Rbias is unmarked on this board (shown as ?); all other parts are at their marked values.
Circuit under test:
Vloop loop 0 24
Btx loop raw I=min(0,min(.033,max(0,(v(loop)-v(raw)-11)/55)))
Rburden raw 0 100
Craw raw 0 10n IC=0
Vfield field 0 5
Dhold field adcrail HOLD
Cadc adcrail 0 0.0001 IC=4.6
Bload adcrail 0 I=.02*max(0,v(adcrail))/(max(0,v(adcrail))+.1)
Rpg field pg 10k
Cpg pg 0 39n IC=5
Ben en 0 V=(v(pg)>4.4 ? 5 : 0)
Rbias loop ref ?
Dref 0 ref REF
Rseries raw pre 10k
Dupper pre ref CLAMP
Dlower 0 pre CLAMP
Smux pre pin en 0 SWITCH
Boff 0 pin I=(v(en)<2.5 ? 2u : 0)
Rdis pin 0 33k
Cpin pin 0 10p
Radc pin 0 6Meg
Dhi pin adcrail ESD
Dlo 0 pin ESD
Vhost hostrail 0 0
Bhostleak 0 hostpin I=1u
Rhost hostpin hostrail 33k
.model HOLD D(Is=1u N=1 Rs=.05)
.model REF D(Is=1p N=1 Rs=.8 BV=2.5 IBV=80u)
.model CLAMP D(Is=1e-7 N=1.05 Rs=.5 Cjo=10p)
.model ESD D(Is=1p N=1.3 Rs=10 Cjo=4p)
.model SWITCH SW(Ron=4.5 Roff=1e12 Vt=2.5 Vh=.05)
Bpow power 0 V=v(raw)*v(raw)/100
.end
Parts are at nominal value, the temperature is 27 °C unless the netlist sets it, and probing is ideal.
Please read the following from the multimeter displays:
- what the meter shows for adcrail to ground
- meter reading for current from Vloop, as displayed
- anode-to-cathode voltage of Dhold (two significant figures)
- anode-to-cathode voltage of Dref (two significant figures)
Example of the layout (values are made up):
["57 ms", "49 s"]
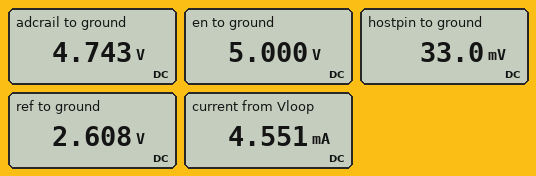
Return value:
["4.743 V", "4.551 mA", "260 mV", "-2.6 V"]
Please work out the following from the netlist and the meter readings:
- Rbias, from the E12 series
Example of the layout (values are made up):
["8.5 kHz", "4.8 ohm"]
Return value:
["4.7 kΩ"]
